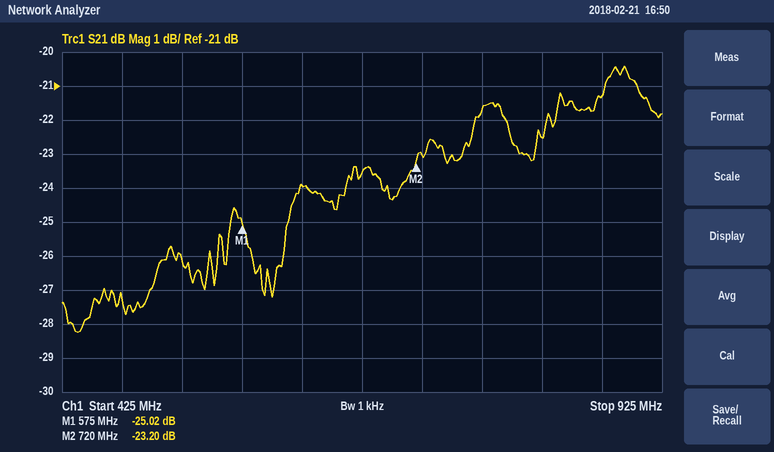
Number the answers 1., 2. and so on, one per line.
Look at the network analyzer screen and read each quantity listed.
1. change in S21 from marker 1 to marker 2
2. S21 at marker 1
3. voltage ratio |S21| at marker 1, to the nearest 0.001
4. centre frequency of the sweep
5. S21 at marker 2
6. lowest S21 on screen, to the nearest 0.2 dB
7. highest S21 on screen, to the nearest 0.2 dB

1. 1.82 dB
2. -25.02 dB
3. 0.056
4. 675 MHz
5. -23.20 dB
6. -28.2 dB
7. -20.4 dB
